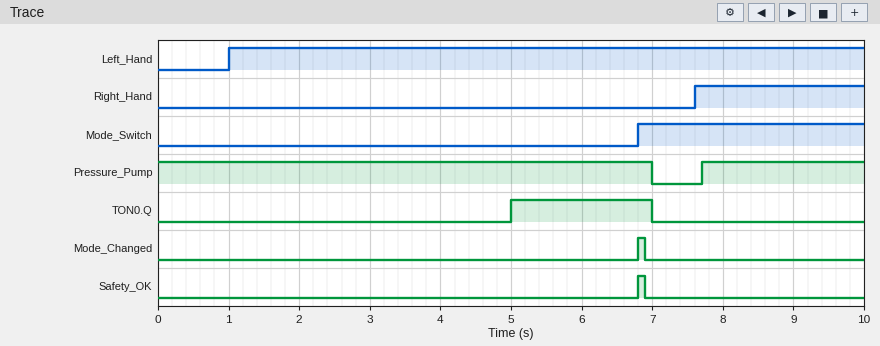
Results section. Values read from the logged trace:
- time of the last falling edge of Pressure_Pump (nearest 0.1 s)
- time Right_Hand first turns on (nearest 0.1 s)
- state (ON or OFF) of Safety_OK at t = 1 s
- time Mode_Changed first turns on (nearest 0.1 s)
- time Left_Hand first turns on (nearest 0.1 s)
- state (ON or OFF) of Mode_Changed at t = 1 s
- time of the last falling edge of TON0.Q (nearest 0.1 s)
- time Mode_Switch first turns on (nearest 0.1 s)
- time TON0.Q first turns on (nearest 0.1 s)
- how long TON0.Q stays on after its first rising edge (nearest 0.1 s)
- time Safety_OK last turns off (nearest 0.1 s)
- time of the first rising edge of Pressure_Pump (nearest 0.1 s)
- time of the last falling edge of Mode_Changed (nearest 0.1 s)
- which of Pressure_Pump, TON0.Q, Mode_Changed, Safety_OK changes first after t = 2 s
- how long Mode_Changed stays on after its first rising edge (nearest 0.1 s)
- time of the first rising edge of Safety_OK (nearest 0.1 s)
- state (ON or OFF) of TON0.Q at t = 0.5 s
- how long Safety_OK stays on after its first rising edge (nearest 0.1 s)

7.0 s
7.6 s
OFF
6.8 s
1.0 s
OFF
7.0 s
6.8 s
5.0 s
2.0 s
6.9 s
7.7 s
6.9 s
TON0.Q
0.1 s
6.8 s
OFF
0.1 s
